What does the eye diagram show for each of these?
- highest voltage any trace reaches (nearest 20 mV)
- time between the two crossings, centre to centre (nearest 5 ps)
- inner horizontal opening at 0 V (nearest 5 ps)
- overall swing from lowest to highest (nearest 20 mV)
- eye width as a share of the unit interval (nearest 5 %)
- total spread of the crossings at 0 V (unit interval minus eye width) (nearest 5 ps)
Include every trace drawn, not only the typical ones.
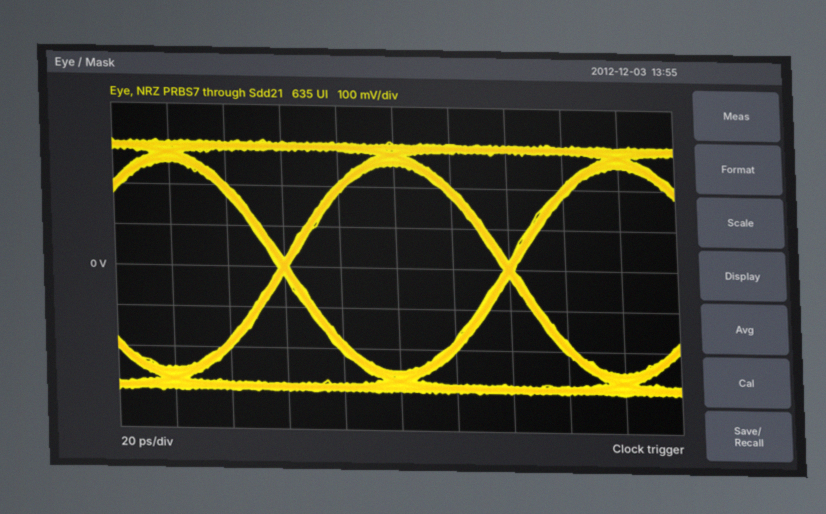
320 mV
80 ps
75 ps
620 mV
95 %
5 ps
